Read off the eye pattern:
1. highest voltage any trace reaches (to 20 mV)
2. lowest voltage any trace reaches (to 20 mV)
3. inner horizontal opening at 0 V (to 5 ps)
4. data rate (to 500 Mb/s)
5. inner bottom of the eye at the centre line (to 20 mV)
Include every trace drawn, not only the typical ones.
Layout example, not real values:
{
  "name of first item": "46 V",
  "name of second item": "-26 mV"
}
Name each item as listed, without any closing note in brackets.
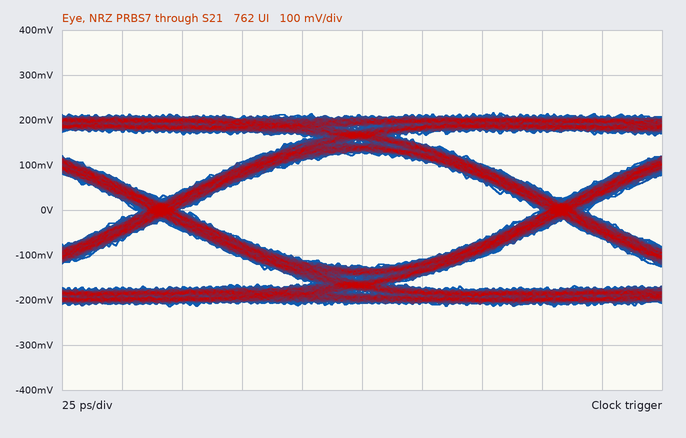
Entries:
{
  "highest voltage any trace reaches": "220 mV",
  "lowest voltage any trace reaches": "-220 mV",
  "inner horizontal opening at 0 V": "150 ps",
  "data rate": "6.0 Gb/s",
  "inner bottom of the eye at the centre line": "-120 mV"
}
